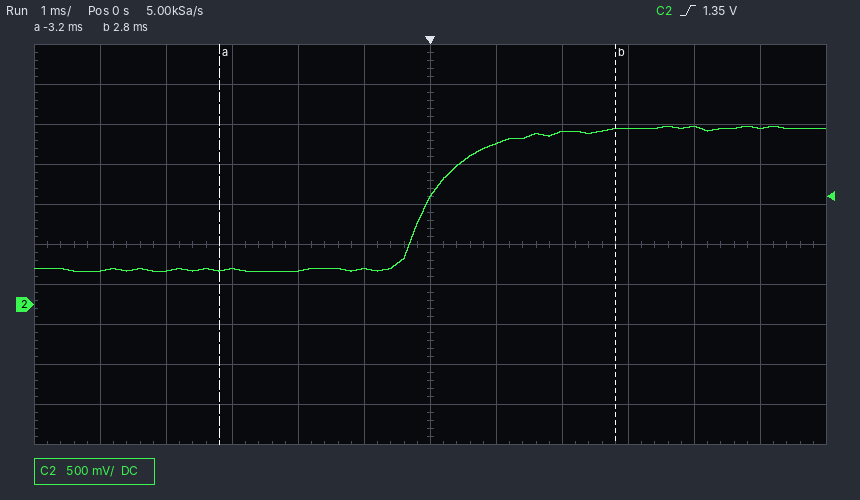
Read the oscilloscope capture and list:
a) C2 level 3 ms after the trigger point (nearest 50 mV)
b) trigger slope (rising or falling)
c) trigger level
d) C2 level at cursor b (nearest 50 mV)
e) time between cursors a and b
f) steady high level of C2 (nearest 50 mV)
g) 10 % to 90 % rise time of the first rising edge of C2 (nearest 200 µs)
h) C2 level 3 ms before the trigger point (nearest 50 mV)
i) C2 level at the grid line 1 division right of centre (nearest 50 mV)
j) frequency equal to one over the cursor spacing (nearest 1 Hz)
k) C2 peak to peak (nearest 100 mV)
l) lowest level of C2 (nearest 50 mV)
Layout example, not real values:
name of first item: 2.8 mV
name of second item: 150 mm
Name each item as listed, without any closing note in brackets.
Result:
C2 level 3 ms after the trigger point: 2.20 V
trigger slope: rising
trigger level: 1.35 V
C2 level at cursor b: 2.20 V
time between cursors a and b: 6.0 ms
steady high level of C2: 2.20 V
10 % to 90 % rise time of the first rising edge of C2: 1.4 ms
C2 level 3 ms before the trigger point: 450 mV
C2 level at the grid line 1 division right of centre: 2.00 V
frequency equal to one over the cursor spacing: 167 Hz
C2 peak to peak: 1.80 V
lowest level of C2: 400 mV
